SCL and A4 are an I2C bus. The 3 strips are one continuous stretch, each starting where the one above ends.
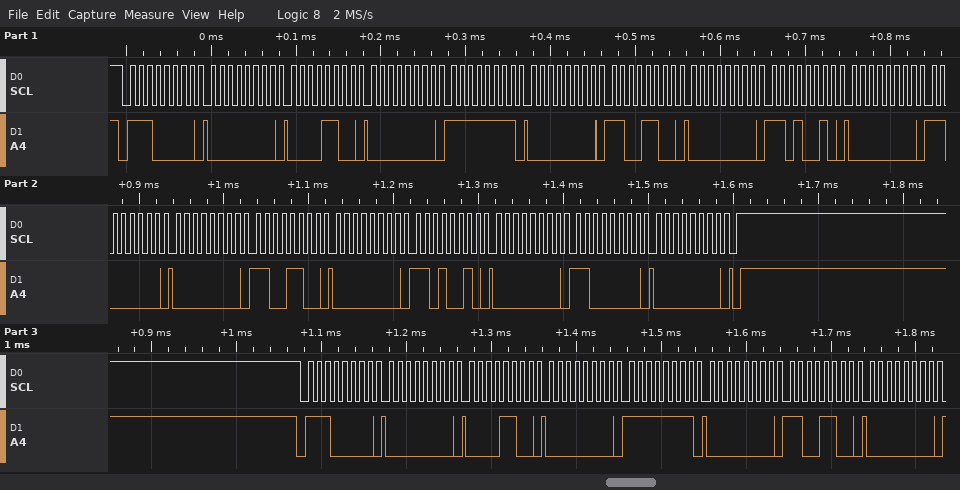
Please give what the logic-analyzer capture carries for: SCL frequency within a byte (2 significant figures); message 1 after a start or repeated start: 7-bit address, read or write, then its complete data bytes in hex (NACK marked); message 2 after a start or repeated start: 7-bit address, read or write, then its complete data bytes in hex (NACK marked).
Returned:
100 kHz
0x70 write: 00 0C 00 FF 00 CC 00 D2 00 C0 00 CC 00 D2 00 C0 00
0x70 write: 00 0C 00 FF 00 CC 00
